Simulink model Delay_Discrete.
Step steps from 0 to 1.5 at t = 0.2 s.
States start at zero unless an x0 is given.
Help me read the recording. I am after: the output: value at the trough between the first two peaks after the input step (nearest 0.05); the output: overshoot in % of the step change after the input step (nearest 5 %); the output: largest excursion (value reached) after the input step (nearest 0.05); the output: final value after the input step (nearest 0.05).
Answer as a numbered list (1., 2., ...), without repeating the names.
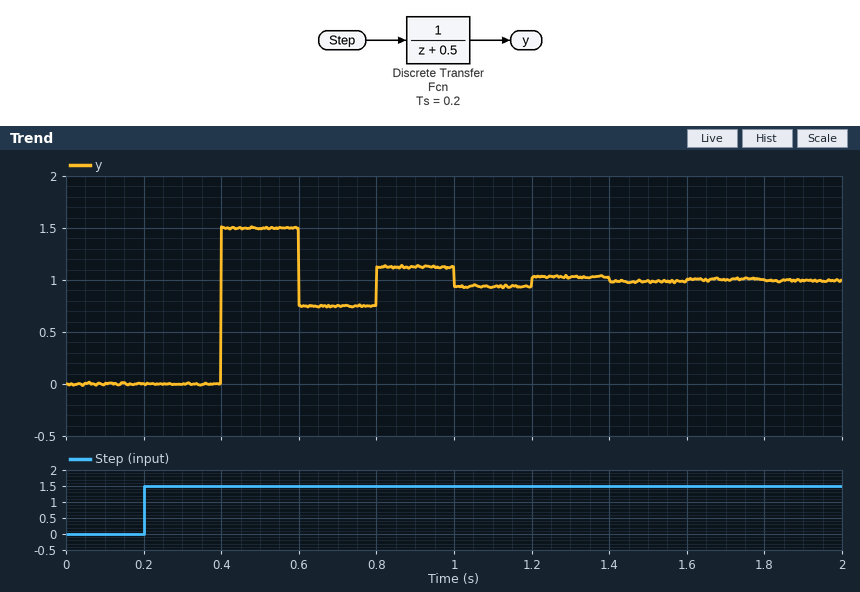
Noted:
1. 0.75
2. 50 %
3. 1.50
4. 1.00
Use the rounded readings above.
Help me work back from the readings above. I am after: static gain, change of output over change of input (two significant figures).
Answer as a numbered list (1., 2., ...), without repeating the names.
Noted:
1. 0.67
